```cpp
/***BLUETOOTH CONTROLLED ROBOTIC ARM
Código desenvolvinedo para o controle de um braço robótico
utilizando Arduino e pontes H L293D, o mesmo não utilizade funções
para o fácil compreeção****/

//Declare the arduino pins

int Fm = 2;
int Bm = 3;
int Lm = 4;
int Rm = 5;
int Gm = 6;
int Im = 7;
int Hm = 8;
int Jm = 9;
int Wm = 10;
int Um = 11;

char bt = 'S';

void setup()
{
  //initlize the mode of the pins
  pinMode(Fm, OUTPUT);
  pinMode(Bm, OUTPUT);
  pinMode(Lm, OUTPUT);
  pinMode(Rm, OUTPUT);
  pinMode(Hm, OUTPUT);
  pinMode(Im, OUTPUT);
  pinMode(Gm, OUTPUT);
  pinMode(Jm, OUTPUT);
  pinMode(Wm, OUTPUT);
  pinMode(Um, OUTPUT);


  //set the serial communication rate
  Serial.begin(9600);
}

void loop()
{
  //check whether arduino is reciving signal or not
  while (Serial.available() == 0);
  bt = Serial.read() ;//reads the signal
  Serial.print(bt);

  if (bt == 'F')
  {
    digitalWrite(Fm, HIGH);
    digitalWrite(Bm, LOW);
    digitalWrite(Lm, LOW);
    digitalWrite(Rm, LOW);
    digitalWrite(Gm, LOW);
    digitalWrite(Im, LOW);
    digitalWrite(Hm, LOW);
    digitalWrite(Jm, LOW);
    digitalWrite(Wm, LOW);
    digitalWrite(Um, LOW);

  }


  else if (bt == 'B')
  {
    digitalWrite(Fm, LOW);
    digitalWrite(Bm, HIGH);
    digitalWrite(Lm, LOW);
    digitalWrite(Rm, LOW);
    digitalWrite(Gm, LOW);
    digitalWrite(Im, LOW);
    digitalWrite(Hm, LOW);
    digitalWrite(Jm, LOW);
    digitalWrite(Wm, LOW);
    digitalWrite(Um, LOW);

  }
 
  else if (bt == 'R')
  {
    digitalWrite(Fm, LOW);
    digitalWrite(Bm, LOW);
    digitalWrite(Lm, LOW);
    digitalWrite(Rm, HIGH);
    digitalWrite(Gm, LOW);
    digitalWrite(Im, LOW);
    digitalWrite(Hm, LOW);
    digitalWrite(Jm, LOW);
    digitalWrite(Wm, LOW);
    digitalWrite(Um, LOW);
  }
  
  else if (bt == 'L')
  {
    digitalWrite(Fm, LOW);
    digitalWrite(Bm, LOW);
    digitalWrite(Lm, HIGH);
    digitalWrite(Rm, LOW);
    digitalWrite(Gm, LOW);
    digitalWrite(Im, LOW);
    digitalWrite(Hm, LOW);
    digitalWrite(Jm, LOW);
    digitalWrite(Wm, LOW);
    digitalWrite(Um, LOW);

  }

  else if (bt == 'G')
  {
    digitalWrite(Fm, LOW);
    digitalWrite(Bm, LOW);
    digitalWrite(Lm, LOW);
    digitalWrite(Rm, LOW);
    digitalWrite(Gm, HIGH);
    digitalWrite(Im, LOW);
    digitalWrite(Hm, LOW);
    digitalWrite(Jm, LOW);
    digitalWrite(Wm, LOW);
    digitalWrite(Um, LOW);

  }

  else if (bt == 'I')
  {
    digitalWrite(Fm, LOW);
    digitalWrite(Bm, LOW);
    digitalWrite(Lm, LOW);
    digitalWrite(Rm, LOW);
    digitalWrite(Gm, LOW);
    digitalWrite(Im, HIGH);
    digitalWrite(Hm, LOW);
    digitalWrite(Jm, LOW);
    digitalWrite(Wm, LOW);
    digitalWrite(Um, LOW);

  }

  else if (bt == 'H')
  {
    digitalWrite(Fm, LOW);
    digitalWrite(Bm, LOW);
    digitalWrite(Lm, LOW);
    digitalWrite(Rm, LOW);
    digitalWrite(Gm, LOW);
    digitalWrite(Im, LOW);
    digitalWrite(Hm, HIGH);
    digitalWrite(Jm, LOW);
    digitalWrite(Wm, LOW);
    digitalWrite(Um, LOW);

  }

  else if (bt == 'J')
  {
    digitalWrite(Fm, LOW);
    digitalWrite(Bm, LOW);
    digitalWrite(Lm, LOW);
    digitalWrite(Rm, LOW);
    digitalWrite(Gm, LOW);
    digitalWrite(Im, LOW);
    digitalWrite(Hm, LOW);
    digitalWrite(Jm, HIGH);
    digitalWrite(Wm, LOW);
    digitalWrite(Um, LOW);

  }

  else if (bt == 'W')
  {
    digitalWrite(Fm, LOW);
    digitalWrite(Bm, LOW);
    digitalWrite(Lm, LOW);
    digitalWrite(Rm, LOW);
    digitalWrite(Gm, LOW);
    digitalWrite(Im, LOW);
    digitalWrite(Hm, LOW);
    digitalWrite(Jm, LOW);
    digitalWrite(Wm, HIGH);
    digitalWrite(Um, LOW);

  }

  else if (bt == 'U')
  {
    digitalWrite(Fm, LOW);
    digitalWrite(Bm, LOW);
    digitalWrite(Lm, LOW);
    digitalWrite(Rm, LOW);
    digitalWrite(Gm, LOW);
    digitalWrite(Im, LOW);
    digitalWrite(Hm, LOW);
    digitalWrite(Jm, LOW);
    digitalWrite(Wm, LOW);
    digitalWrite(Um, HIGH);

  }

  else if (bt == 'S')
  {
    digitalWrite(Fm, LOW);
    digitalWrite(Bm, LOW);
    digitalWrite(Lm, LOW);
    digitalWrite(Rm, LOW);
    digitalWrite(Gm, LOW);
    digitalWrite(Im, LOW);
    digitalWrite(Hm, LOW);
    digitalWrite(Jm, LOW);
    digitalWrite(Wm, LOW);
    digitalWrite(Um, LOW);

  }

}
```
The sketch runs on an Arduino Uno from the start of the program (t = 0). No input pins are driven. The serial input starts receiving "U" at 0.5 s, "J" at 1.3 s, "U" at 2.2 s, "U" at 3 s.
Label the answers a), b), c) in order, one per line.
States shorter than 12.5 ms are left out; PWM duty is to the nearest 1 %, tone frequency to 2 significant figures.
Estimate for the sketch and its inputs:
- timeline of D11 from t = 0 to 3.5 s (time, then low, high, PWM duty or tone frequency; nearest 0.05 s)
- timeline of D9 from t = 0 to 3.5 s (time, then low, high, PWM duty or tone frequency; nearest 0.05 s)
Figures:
a) 0 s low; 0.5 s high; 1.3 s low; 2.2 s high
b) 0 s low; 1.3 s high; 2.2 s low
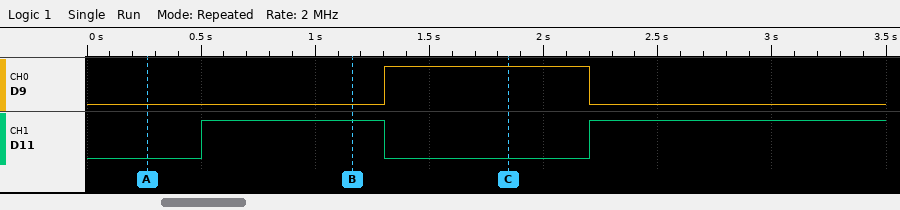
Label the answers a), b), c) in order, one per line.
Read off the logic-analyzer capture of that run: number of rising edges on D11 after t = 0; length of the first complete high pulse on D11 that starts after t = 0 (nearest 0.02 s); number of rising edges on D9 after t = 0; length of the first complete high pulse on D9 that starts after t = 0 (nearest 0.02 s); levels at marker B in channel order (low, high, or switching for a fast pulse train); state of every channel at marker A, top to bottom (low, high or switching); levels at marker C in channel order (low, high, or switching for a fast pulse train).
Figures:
a) 2
b) 0.80 s
c) 1
d) 0.90 s
e) D9 low, D11 high
f) D9 low, D11 low
g) D9 high, D11 low
